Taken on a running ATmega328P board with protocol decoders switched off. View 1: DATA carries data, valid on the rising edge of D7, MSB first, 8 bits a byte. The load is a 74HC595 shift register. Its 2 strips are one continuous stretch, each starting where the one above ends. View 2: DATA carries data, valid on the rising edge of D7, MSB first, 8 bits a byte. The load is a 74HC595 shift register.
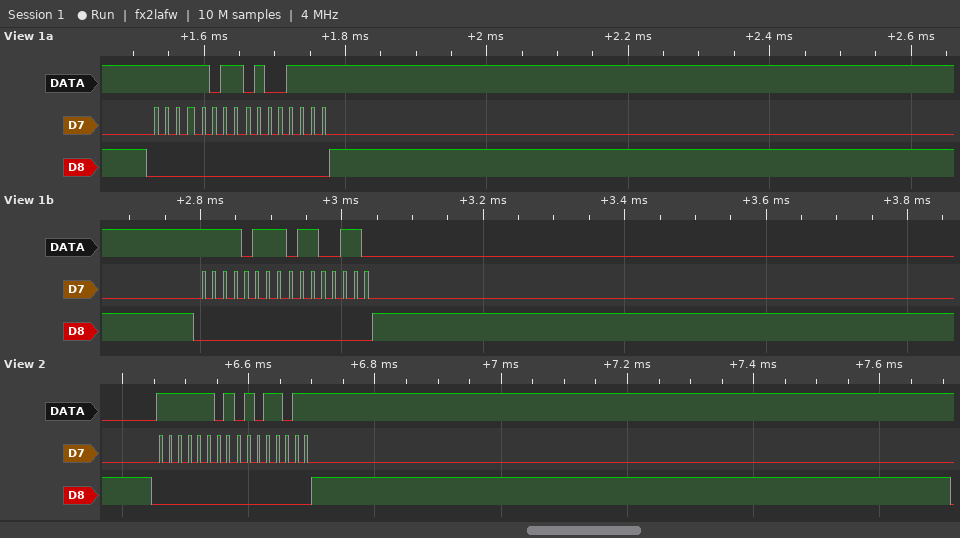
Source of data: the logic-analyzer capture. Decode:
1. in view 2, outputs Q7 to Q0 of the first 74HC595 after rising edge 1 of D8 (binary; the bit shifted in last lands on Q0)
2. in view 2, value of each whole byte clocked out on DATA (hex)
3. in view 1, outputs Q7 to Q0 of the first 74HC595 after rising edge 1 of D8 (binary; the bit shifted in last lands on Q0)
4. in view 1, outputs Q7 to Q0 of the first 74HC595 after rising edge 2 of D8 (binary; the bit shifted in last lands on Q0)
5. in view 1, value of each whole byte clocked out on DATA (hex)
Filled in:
01011011
FD 5B
01001111
01100110
0xFB 0x4F 0xF7 0x66
